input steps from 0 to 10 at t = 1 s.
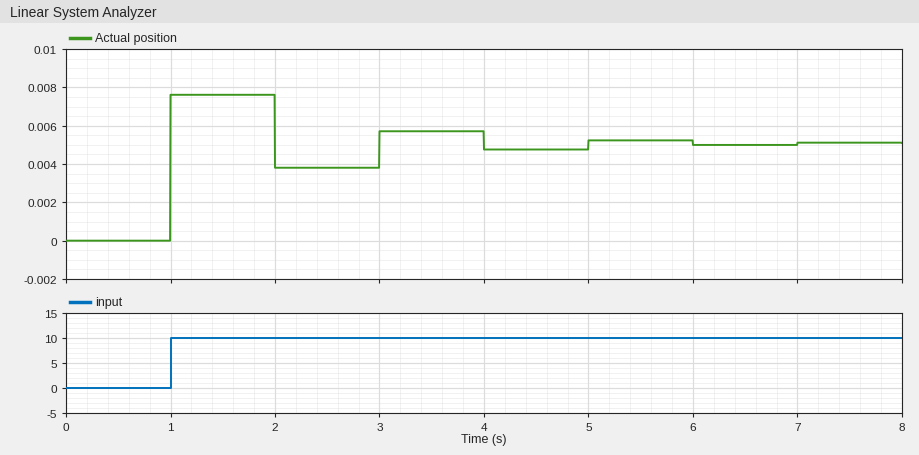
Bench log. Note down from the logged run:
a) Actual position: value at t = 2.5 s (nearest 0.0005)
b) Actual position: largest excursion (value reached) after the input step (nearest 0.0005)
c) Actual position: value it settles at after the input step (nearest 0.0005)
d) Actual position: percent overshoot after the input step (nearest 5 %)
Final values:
0.0040
0.0075
0.0050
50 %
